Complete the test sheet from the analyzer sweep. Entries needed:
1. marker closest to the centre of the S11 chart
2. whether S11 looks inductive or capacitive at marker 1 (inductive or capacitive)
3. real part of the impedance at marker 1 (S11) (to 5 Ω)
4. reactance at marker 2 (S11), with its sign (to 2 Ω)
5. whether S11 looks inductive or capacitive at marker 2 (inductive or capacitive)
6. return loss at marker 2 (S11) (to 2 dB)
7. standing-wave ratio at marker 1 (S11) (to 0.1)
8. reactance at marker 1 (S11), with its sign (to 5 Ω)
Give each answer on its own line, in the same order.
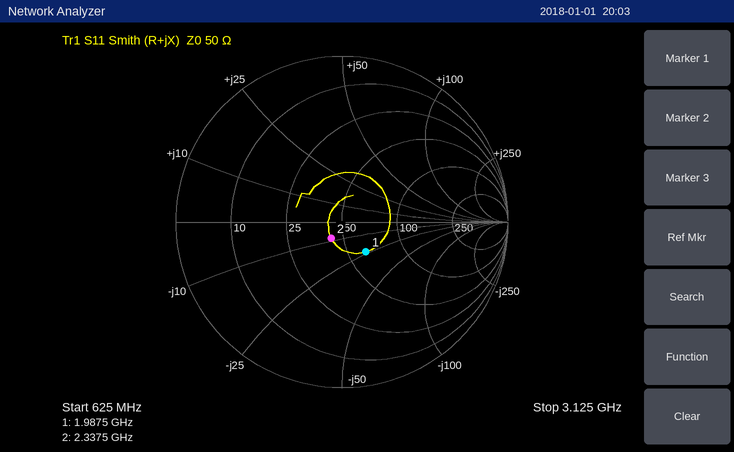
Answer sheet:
marker 2
capacitive
60 Ω
-8 Ω
capacitive
18 dB
1.6
-25 Ω
